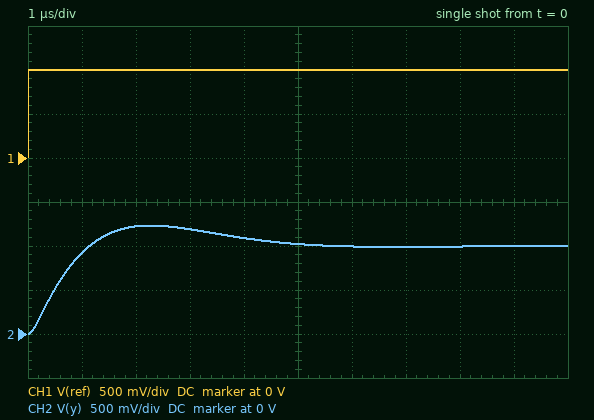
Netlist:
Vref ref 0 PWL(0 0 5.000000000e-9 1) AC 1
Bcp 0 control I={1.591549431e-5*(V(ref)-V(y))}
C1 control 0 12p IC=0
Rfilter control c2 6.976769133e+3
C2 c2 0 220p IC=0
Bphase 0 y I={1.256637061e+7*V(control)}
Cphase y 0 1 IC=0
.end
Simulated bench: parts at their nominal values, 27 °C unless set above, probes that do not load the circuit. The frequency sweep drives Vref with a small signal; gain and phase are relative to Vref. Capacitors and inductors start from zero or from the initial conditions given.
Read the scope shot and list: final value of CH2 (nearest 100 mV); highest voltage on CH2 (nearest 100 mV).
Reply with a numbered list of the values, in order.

1. 1.0 V
2. 1.2 V
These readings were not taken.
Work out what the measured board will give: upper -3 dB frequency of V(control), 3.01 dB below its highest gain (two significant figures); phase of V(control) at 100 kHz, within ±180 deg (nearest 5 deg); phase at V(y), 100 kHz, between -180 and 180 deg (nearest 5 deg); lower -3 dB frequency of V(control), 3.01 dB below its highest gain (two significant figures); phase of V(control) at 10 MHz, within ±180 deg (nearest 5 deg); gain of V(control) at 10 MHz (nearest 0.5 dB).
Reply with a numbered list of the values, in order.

1. 1.8 MHz
2. 75 deg
3. -15 deg
4. 130 kHz
5. -80 deg
6. -33.5 dB
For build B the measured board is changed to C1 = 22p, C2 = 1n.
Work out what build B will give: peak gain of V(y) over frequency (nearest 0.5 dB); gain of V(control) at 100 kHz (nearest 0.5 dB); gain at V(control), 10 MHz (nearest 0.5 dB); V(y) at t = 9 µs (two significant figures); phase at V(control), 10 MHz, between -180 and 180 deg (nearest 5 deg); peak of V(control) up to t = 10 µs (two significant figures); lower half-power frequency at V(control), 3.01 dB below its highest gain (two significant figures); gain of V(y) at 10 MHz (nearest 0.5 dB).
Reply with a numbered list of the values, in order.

1. 0.5 dB
2. -25.5 dB
3. -39.0 dB
4. 1.0 V
5. -85 deg
6. 85 mV
7. 170 kHz
8. -53.0 dB
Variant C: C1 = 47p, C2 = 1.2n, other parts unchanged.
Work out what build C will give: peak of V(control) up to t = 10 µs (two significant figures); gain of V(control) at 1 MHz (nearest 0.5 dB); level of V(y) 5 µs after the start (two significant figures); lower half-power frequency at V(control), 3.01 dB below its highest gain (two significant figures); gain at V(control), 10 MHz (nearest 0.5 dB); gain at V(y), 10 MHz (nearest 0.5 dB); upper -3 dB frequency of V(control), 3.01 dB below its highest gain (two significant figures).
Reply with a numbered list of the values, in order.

1. 74 mV
2. -25.5 dB
3. 1.1 V
4. 150 kHz
5. -45.5 dB
6. -59.5 dB
7. 640 kHz
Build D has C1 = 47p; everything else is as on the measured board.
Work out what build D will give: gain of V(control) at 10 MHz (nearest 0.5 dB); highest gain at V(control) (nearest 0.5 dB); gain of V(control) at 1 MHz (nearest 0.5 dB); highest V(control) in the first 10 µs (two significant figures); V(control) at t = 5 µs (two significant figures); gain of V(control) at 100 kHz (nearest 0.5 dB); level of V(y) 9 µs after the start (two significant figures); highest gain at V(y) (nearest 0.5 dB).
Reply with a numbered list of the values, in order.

1. -45.5 dB
2. -17.5 dB
3. -26.0 dB
4. 81 mV
5. -5.4 mV
6. -23.0 dB
7. 1.0 V
8. 3.5 dB
